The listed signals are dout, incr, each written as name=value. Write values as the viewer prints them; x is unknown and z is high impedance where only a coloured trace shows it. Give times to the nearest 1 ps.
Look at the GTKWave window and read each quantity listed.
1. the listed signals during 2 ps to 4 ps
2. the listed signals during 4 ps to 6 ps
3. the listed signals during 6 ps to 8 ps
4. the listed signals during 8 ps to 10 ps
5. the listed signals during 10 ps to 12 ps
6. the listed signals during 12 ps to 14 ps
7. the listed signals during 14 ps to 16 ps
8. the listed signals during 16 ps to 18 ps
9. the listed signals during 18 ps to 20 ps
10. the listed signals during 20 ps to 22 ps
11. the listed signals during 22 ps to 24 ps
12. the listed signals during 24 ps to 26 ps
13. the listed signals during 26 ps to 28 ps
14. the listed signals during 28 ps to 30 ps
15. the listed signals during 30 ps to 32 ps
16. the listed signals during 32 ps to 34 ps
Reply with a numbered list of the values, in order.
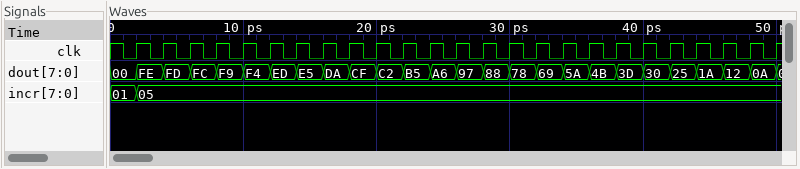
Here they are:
1. dout=FE, incr=05
2. dout=FD, incr=05
3. dout=FC, incr=05
4. dout=F9, incr=05
5. dout=F4, incr=05
6. dout=ED, incr=05
7. dout=E5, incr=05
8. dout=DA, incr=05
9. dout=CF, incr=05
10. dout=C2, incr=05
11. dout=B5, incr=05
12. dout=A6, incr=05
13. dout=97, incr=05
14. dout=88, incr=05
15. dout=78, incr=05
16. dout=69, incr=05
